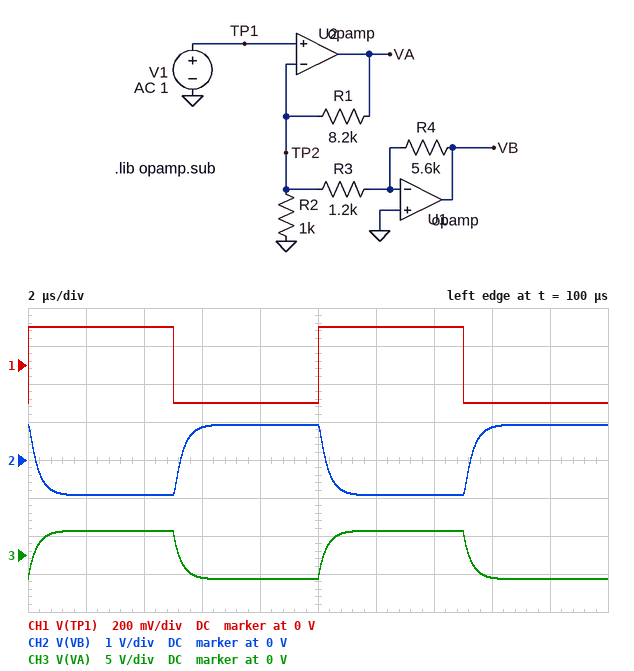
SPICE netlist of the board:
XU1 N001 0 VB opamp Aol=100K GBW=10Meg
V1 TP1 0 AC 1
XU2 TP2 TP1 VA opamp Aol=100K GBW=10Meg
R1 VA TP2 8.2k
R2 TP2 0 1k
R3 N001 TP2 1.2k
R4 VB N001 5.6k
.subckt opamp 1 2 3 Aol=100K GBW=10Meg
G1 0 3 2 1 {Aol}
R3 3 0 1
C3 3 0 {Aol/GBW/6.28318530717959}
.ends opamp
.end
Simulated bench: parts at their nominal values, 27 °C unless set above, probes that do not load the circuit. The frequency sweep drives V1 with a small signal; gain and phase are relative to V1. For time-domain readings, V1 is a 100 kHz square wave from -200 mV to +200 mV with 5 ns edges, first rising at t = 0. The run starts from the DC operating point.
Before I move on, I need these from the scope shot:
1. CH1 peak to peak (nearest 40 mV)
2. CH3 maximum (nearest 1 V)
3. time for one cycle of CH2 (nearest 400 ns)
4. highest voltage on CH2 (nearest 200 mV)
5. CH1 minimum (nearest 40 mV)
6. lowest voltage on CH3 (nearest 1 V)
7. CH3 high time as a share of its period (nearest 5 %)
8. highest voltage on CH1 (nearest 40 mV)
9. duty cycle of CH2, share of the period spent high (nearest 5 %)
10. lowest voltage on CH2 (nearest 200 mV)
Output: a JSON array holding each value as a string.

["400 mV", "3 V", "10.0 µs", "1.0 V", "-200 mV", "-3 V", "50 %", "200 mV", "50 %", "-1.0 V"]
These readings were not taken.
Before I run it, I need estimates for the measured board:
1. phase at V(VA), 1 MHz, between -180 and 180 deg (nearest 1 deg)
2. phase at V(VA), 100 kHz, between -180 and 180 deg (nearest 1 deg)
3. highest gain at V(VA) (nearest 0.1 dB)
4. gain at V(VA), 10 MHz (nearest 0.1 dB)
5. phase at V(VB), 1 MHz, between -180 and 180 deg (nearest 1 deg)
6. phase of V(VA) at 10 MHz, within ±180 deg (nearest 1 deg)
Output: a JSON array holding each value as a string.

["-59 deg", "-10 deg", "24.1 dB", "-0.1 dB", "101 deg", "-85 deg"]
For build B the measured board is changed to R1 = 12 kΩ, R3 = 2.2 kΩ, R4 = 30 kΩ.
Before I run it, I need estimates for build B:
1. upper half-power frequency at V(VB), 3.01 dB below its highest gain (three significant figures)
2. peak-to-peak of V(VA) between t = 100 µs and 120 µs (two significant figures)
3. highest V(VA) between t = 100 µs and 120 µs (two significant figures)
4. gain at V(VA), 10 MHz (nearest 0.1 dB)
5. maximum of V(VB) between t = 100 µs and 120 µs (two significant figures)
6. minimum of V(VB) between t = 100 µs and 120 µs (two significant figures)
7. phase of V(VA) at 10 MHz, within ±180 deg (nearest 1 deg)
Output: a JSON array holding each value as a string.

["364 kHz", "7.4 V", "3.7 V", "0 dB", "2.7 V", "-2.7 V", "-86 deg"]
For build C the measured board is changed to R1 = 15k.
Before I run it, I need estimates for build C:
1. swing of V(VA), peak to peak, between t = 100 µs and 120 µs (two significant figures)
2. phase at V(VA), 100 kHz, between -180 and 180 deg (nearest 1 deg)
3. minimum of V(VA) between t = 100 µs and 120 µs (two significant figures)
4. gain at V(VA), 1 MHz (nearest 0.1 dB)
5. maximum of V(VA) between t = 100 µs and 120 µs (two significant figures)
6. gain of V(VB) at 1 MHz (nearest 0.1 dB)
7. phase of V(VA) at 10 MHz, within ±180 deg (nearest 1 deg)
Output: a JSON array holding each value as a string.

["11 V", "-17 deg", "-5.7 V", "19.0 dB", "5.7 V", "2.7 dB", "-87 deg"]
